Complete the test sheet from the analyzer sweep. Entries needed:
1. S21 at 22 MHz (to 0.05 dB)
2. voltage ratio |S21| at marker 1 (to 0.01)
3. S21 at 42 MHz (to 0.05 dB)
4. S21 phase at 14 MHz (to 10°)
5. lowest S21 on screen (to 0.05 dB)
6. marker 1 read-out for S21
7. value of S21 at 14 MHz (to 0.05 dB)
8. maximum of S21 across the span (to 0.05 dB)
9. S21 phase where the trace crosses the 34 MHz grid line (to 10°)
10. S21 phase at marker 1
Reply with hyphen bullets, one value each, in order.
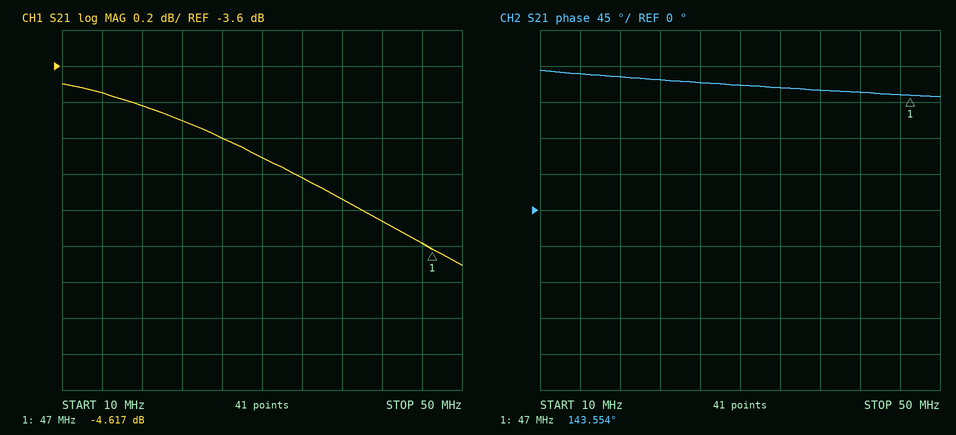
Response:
- -3.90 dB
- 0.59
- -4.45 dB
- 170°
- -4.70 dB
- -4.617 dB
- -3.75 dB
- -3.70 dB
- 150°
- 143.554°
